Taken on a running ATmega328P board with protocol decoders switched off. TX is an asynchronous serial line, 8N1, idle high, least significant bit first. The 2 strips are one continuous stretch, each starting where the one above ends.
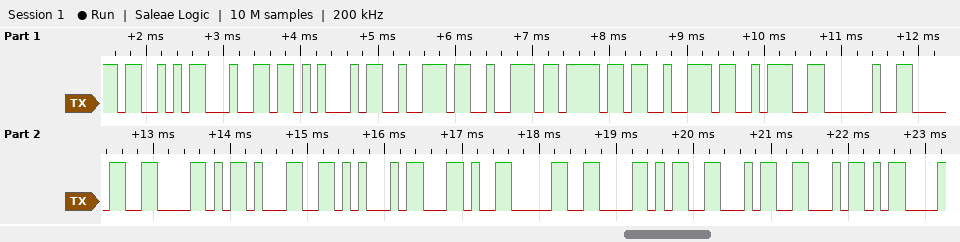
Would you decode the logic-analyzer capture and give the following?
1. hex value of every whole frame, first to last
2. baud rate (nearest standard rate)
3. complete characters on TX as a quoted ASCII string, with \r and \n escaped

53 64 45 72 72 6F 72 3A 20 30 58 31 45 2C 30 58 46 46 0D
9600 baud
"SdError: 0X1E,0XFF\r"
